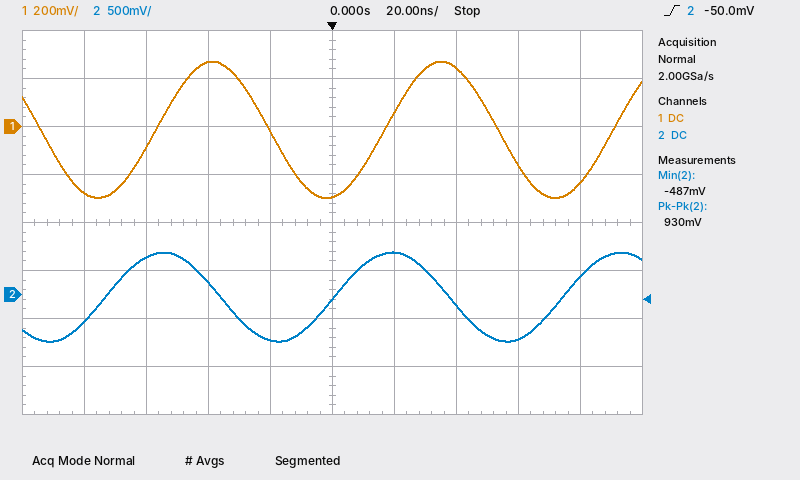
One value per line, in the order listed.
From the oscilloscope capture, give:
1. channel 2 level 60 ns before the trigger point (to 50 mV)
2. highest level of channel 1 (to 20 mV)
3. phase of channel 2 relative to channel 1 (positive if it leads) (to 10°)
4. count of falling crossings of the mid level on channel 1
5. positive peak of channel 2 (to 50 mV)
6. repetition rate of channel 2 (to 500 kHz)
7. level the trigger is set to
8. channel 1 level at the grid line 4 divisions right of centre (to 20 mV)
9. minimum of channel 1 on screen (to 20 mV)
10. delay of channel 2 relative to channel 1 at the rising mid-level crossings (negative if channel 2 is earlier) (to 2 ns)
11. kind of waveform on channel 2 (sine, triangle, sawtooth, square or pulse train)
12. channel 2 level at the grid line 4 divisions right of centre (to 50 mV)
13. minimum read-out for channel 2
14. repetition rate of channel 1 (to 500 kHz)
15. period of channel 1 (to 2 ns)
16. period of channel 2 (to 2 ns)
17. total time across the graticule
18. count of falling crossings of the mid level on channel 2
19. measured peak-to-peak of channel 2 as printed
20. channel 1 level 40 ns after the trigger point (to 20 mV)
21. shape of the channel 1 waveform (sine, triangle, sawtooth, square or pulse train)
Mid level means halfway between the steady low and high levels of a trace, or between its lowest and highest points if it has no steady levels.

400 mV
280 mV
+80°
3
450 mV
13.5 MHz
-50.0 mV
-240 mV
-300 mV
-16 ns
sine
200 mV
-487 mV
13.5 MHz
74 ns
74 ns
200 ns
2
930 mV
240 mV
sine
